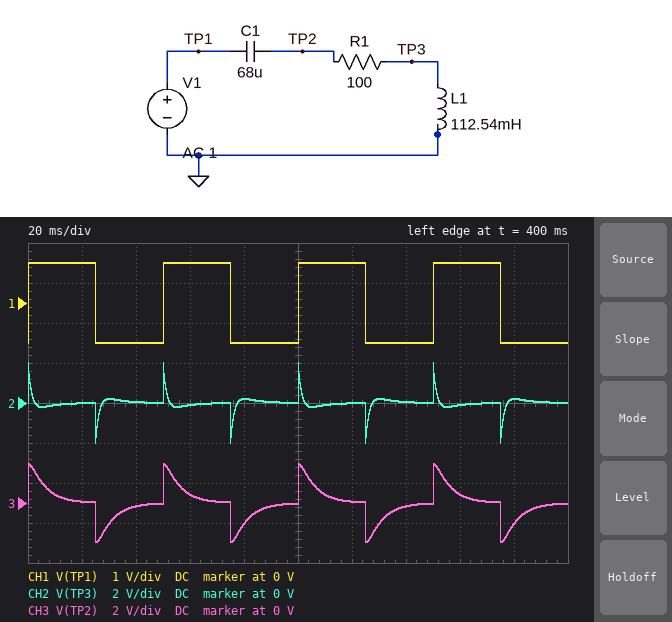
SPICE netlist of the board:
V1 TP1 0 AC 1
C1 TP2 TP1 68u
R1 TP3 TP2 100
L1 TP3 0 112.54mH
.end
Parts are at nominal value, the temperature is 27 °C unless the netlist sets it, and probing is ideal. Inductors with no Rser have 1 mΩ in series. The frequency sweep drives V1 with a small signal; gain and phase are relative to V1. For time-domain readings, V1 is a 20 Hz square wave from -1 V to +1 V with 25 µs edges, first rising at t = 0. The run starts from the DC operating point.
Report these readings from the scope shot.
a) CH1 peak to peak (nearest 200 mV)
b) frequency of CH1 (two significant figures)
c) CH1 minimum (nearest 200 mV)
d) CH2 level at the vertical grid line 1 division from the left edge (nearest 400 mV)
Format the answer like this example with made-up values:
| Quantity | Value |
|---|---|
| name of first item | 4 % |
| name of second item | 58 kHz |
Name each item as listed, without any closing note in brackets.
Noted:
| Quantity | Value |
|---|---|
| CH1 peak to peak | 2.0 V |
| frequency of CH1 | 20 Hz |
| CH1 minimum | -1.0 V |
| CH2 level at the vertical grid line 1 division from the left edge | 0 V |
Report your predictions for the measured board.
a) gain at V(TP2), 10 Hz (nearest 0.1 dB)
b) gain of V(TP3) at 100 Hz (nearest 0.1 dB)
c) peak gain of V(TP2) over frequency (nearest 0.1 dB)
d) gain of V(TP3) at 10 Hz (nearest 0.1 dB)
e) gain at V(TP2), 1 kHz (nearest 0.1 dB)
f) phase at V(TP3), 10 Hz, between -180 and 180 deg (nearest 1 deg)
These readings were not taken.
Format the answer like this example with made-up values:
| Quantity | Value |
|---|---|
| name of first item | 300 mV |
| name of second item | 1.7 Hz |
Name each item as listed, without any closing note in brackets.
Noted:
| Quantity | Value |
|---|---|
| gain at V(TP2), 10 Hz | -7.9 dB |
| gain of V(TP3) at 100 Hz | -3.9 dB |
| peak gain of V(TP2) over frequency | 0.9 dB |
| gain of V(TP3) at 10 Hz | -30.9 dB |
| gain at V(TP2), 1 kHz | 0 dB |
| phase at V(TP3), 10 Hz, between -180 and 180 deg | 156 deg |
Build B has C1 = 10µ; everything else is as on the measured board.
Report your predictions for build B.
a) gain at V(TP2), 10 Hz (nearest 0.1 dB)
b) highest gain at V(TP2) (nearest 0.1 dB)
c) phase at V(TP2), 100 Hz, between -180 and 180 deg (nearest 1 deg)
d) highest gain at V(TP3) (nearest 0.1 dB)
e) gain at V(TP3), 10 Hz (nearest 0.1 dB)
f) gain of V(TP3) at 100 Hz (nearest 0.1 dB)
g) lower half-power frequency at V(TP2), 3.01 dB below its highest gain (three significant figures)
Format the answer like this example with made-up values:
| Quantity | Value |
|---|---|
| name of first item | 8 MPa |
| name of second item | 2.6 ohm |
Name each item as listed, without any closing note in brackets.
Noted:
| Quantity | Value |
|---|---|
| gain at V(TP2), 10 Hz | -24.0 dB |
| highest gain at V(TP2) | 3.6 dB |
| phase at V(TP2), 100 Hz, between -180 and 180 deg | 77 deg |
| highest gain at V(TP3) | 1.6 dB |
| gain at V(TP3), 10 Hz | -47.0 dB |
| gain of V(TP3) at 100 Hz | -5.5 dB |
| lower half-power frequency at V(TP2), 3.01 dB below its highest gain | 111 Hz |
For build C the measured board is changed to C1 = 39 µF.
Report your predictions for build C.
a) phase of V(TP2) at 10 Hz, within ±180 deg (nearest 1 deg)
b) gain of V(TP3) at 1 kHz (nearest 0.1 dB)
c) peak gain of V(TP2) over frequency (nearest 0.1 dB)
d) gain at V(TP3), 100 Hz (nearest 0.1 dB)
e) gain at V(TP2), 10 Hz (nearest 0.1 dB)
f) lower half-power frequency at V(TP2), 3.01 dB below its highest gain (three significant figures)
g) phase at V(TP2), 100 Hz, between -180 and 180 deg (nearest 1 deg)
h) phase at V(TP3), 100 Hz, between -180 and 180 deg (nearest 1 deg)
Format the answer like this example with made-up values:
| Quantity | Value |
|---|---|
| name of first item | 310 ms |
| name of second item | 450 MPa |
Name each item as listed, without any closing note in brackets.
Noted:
| Quantity | Value |
|---|---|
| phase of V(TP2) at 10 Hz, within ±180 deg | 80 deg |
| gain of V(TP3) at 1 kHz | 0 dB |
| peak gain of V(TP2) over frequency | 1.4 dB |
| gain at V(TP3), 100 Hz | -3.4 dB |
| gain at V(TP2), 10 Hz | -12.3 dB |
| lower half-power frequency at V(TP2), 3.01 dB below its highest gain | 39.6 Hz |
| phase at V(TP2), 100 Hz, between -180 and 180 deg | 19 deg |
| phase at V(TP3), 100 Hz, between -180 and 180 deg | 73 deg |
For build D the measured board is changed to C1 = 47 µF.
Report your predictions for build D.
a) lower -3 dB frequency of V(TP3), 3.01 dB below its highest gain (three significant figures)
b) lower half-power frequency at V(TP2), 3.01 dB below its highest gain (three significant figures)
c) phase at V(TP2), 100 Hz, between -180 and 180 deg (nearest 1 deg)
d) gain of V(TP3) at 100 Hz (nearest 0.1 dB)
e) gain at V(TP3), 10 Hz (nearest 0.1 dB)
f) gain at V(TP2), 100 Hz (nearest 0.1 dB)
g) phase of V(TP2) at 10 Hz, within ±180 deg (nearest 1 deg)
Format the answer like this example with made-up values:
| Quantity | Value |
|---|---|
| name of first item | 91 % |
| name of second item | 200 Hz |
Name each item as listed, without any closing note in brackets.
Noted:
| Quantity | Value |
|---|---|
| lower -3 dB frequency of V(TP3), 3.01 dB below its highest gain | 111 Hz |
| lower half-power frequency at V(TP2), 3.01 dB below its highest gain | 33.5 Hz |
| phase at V(TP2), 100 Hz, between -180 and 180 deg | 15 deg |
| gain of V(TP3) at 100 Hz | -3.6 dB |
| gain at V(TP3), 10 Hz | -33.8 dB |
| gain at V(TP2), 100 Hz | 1.2 dB |
| phase of V(TP2) at 10 Hz, within ±180 deg | 77 deg |
